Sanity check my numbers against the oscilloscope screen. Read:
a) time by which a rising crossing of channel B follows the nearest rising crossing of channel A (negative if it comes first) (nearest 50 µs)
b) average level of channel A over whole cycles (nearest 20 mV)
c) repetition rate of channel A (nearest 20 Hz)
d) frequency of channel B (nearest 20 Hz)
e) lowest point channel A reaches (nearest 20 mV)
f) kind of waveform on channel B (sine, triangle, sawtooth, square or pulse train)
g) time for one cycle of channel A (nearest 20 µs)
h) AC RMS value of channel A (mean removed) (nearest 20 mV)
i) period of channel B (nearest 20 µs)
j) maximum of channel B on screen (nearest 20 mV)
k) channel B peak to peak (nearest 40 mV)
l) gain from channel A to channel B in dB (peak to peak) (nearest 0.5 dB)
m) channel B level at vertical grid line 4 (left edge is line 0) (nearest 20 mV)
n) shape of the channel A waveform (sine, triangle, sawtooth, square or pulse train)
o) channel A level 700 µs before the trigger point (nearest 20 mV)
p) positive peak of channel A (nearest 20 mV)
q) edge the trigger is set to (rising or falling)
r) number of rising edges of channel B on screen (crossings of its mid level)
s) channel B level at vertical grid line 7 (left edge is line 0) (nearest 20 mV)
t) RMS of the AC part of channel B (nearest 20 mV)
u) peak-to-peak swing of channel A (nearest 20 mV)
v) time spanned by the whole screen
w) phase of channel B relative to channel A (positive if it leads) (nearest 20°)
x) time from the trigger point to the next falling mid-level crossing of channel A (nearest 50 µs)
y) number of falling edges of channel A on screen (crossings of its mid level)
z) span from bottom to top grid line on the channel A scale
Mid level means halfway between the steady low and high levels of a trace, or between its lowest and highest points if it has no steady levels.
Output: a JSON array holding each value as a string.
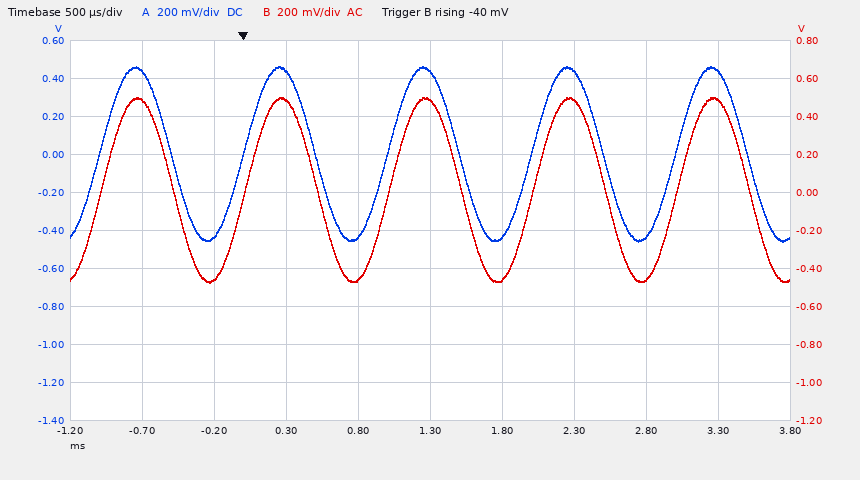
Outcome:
["0 µs", "0 mV", "1.00 kHz", "1.00 kHz", "-460 mV", "sine", "1.00 ms", "320 mV", "1.00 ms", "500 mV", "960 mV", "0.5 dB", "-460 mV", "sine", "440 mV", "460 mV", "rising", "5", "480 mV", "340 mV", "920 mV", "5 ms", "0°", "500 µs", "5", "2 V"]
